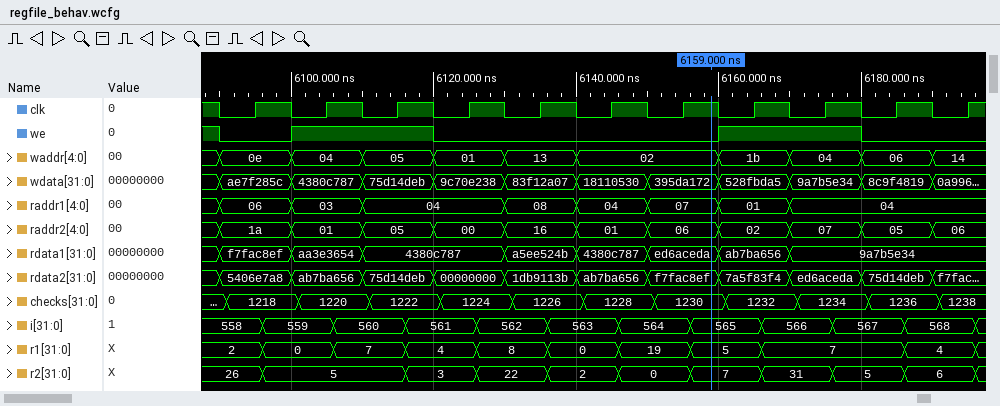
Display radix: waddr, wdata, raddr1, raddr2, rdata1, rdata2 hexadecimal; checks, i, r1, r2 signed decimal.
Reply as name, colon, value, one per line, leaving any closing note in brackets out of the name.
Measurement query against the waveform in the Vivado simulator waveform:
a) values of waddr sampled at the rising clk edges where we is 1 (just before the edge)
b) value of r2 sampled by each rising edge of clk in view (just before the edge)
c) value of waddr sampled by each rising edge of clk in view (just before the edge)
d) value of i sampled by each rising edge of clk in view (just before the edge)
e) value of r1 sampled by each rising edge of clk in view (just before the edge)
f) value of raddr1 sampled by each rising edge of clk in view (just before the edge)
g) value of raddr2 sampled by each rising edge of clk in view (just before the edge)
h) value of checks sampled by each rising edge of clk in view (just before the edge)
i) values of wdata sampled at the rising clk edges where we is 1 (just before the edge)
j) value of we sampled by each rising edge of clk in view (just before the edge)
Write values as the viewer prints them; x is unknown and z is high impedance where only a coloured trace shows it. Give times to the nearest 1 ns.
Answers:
values of waddr sampled at the rising clk edges where we is 1: 04, 05, 1b, 04
value of r2 sampled by each rising edge of clk in view: 26, 5, 5, 3, 22, 2, 0, 7, 31, 5, 6
value of waddr sampled by each rising edge of clk in view: 0e, 04, 05, 01, 13, 02, 02, 1b, 04, 06, 14
value of i sampled by each rising edge of clk in view: 558, 559, 560, 561, 562, 563, 564, 565, 566, 567, 568
value of r1 sampled by each rising edge of clk in view: 2, 0, 7, 4, 8, 0, 19, 5, 7, 7, 4
value of raddr1 sampled by each rising edge of clk in view: 06, 03, 04, 04, 08, 04, 07, 01, 04, 04, 04
value of raddr2 sampled by each rising edge of clk in view: 1a, 01, 05, 00, 16, 01, 06, 02, 07, 05, 06
value of checks sampled by each rising edge of clk in view: 1218, 1220, 1222, 1224, 1226, 1228, 1230, 1232, 1234, 1236, 1238
values of wdata sampled at the rising clk edges where we is 1: 4380c787, 75d14deb, 528fbda5, 9a7b5e34
value of we sampled by each rising edge of clk in view: 0 1 1 0 0 0 0 1 1 0 0
